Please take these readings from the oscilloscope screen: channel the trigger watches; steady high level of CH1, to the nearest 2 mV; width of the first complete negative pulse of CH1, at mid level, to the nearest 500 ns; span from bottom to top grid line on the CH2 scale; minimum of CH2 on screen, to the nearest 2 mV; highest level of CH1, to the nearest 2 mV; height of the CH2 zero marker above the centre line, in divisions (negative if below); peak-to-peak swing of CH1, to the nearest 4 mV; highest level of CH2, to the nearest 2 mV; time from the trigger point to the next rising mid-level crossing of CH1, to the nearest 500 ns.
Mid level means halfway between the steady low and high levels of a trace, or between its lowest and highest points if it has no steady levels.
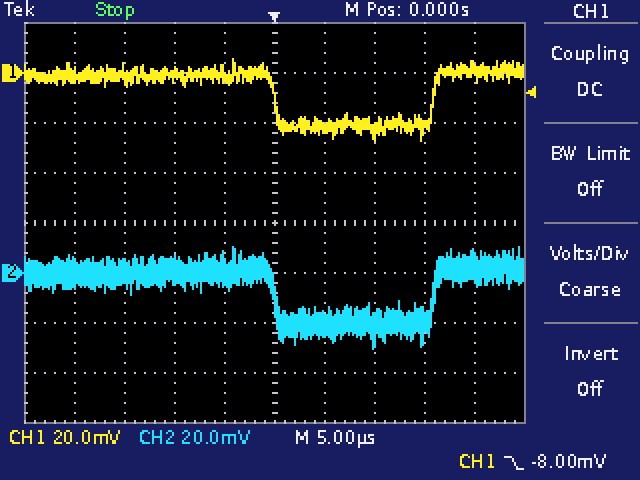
CH1
0 mV
16.0 µs
160 mV
-30 mV
6 mV
-1.0 div
32 mV
10 mV
16.0 µs
